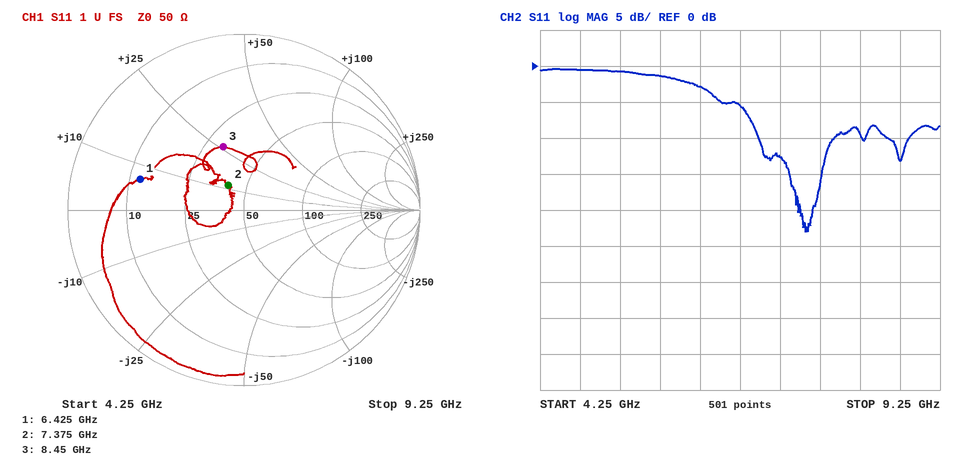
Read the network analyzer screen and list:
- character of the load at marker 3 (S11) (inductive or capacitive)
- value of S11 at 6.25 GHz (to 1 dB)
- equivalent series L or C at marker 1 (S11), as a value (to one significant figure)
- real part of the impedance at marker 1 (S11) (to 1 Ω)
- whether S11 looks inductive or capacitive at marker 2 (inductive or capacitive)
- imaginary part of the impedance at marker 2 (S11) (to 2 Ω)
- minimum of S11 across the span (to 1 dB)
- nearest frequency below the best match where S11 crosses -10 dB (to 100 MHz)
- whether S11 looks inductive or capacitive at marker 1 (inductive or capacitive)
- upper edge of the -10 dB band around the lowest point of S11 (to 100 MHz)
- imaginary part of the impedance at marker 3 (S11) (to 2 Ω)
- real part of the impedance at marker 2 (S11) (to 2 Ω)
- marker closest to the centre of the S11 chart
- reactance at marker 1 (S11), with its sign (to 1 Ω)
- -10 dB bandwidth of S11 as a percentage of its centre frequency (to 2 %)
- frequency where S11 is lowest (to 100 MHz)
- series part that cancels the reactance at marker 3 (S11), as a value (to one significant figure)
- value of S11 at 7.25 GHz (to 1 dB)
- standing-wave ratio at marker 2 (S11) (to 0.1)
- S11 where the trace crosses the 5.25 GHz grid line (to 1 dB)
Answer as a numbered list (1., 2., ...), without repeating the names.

1. inductive
2. -3 dB
3. 200 pH
4. 12 Ω
5. inductive
6. +12 Ω
7. -23 dB
8. 7.0 GHz
9. inductive
10. 7.9 GHz
11. +26 Ω
12. 40 Ω
13. marker 2
14. +7 Ω
15. 12 %
16. 7.6 GHz
17. 700 fF
18. -13 dB
19. 1.4
20. -1 dB
